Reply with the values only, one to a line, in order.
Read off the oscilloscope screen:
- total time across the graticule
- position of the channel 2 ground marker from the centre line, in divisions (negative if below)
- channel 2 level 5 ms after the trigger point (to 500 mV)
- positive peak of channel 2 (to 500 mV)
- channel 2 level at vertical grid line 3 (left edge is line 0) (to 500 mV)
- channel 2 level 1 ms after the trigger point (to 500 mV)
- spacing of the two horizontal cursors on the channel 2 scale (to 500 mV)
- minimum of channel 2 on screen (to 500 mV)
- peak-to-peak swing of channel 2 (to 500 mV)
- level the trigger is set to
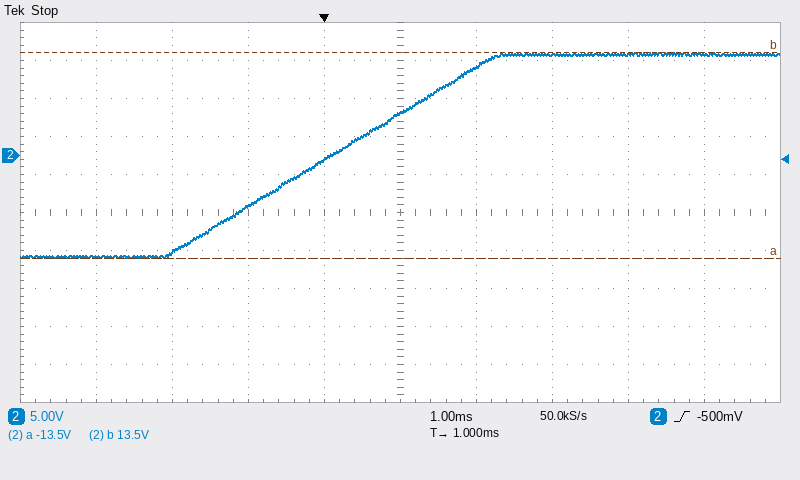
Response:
10 ms
+1.5 div
13.5 V
13.5 V
-6.5 V
5.5 V
27.0 V
-13.5 V
27.0 V
-500 mV
